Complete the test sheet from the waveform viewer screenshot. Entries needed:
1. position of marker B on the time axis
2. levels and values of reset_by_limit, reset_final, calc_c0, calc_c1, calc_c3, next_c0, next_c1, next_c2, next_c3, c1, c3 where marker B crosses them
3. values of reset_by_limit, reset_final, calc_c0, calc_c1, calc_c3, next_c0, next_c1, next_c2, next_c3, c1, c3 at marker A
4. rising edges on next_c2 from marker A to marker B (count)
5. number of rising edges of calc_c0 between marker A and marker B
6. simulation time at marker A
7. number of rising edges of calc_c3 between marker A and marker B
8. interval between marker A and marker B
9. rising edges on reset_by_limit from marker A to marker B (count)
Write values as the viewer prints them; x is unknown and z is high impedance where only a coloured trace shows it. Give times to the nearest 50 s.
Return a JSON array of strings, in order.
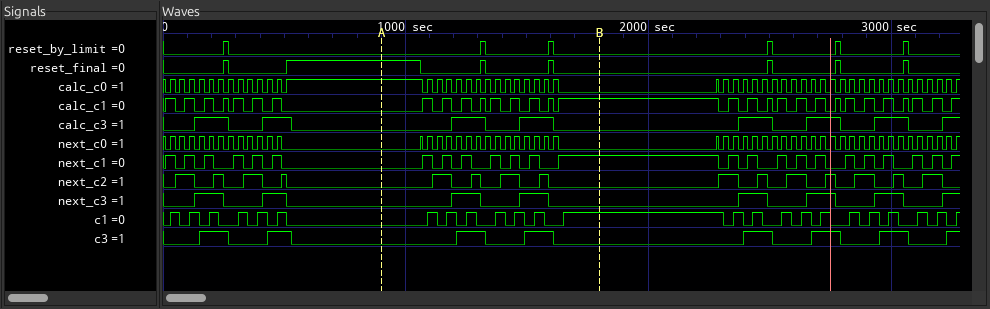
["1800 s", "reset_by_limit=0, reset_final=0, calc_c0=0, calc_c1=1, calc_c3=0, next_c0=0, next_c1=1, next_c2=0, next_c3=0, c1=1, c3=0", "reset_by_limit=0, reset_final=1, calc_c0=1, calc_c1=0, calc_c3=0, next_c0=0, next_c1=0, next_c2=0, next_c3=0, c1=0, c3=0", "4", "14", "900 s", "2", "900 s", "2"]
